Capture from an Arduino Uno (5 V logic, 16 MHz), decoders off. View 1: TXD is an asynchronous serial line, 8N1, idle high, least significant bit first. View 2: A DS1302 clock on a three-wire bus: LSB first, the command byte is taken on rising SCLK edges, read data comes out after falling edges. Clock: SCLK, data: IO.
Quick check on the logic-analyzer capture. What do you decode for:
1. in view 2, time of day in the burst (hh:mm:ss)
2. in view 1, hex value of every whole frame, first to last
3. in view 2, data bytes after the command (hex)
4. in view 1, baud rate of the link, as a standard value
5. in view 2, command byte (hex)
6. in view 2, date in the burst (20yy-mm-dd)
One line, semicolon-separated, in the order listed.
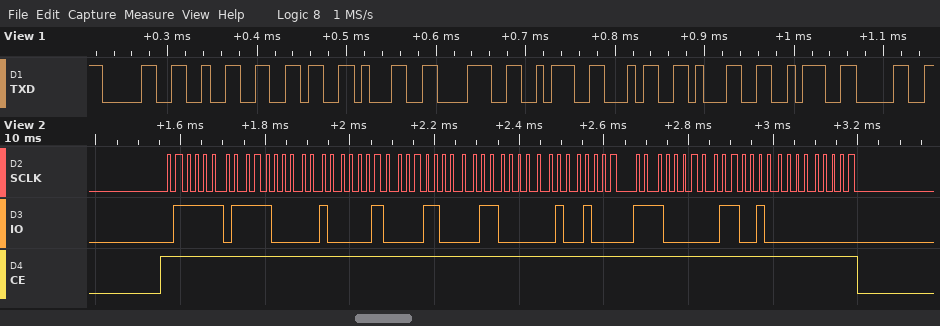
18:41:07; 30 32 36 31 38 3A 34 31 3A 30; 07 41 18 06 12 07 26 00; 115200 baud; 0xBE; 2026-12-06
